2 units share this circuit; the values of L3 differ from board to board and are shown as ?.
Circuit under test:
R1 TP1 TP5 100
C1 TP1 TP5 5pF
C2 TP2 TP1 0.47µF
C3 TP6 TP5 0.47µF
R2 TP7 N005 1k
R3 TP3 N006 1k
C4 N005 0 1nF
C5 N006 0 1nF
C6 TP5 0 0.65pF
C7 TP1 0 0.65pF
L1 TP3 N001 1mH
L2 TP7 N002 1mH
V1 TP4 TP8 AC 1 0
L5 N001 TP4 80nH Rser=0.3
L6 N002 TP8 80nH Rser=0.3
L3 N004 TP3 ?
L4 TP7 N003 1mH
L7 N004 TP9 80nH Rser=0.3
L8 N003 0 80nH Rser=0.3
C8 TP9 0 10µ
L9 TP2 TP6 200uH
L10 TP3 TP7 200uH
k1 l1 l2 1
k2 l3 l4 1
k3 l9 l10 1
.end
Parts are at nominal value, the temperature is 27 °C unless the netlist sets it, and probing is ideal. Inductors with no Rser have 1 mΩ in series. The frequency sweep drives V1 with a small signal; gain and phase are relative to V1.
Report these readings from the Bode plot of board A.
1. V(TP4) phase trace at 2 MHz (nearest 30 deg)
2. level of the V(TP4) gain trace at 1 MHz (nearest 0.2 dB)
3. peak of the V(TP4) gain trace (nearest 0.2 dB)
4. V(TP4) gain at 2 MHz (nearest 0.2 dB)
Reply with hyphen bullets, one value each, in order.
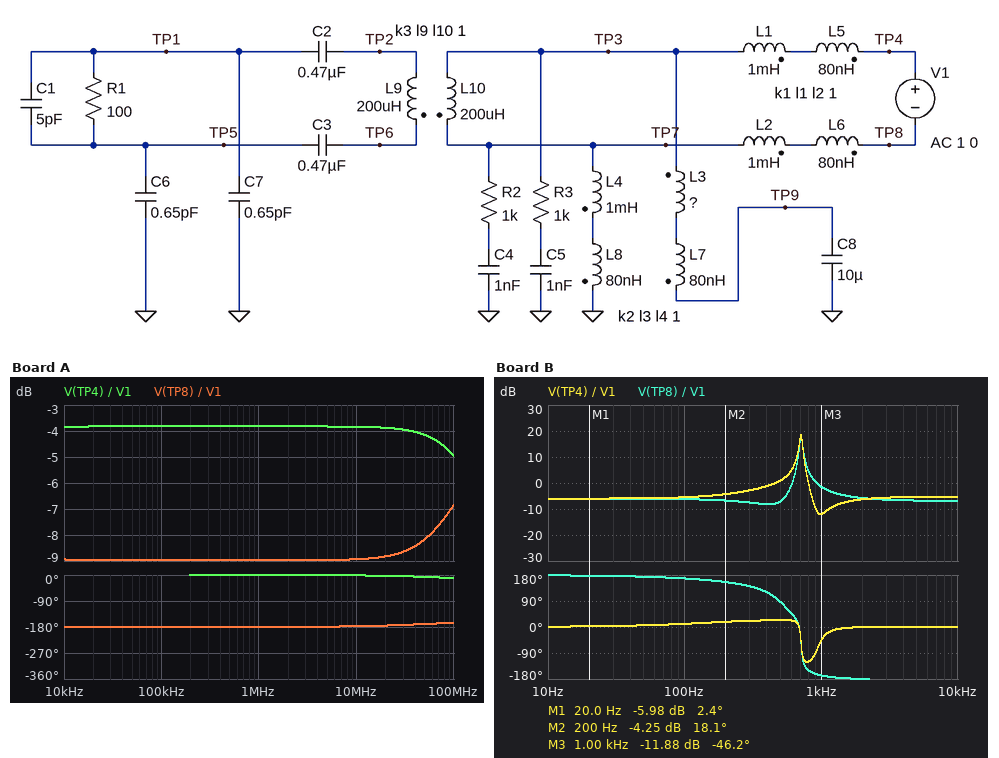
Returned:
- 0 deg
- -3.8 dB
- -3.8 dB
- -3.8 dB
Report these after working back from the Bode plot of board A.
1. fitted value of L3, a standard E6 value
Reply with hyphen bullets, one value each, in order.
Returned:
- 3.3 mH
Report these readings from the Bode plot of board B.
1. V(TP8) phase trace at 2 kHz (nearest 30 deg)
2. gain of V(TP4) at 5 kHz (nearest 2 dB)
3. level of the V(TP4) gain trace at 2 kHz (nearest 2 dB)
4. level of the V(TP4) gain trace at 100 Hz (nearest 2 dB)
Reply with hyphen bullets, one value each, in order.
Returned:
- -180 deg
- -6 dB
- -6 dB
- -6 dB
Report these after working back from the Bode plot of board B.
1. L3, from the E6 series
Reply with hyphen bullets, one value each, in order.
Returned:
- 1.5 mH
